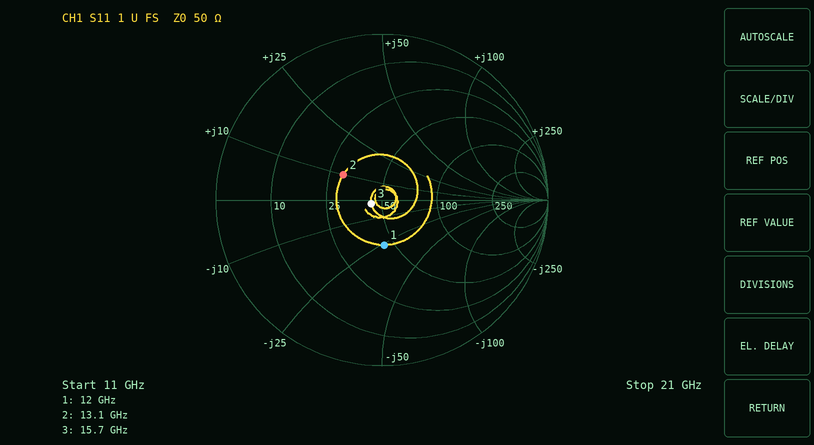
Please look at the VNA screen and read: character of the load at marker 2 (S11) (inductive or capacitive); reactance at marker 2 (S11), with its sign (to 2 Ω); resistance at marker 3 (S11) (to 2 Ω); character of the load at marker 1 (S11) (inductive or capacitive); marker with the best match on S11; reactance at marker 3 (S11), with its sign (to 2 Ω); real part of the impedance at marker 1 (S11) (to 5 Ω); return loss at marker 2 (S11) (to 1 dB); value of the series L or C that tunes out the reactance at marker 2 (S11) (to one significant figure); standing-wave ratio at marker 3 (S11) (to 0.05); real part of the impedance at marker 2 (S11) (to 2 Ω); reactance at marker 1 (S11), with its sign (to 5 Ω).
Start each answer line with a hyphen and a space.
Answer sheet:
- inductive
- +10 Ω
- 44 Ω
- capacitive
- marker 3
- -2 Ω
- 45 Ω
- 11 dB
- 1 pF
- 1.15
- 30 Ω
- -25 Ω
